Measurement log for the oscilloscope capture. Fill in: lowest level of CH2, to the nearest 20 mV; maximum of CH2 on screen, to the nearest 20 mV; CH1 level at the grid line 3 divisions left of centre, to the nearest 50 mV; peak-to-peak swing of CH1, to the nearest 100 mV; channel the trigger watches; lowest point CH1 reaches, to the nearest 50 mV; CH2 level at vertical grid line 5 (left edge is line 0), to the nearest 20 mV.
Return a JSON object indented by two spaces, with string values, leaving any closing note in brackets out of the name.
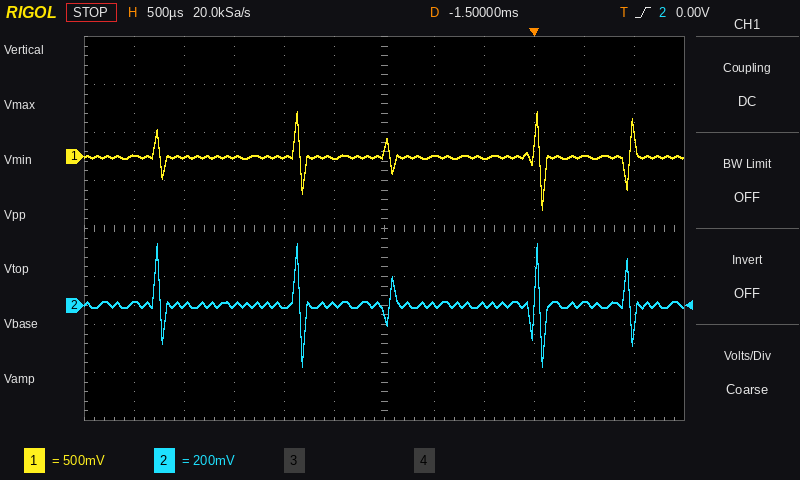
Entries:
{
  "lowest level of CH2, to the nearest 20 mV": "-260 mV",
  "maximum of CH2 on screen, to the nearest 20 mV": "260 mV",
  "CH1 level at the grid line 3 divisions left of centre, to the nearest 50 mV": "0 mV",
  "peak-to-peak swing of CH1, to the nearest 100 mV": "1.00 V",
  "channel the trigger watches": "CH2",
  "lowest point CH1 reaches, to the nearest 50 mV": "-550 mV",
  "CH2 level at vertical grid line 5 (left edge is line 0), to the nearest 20 mV": "0 mV"
}
